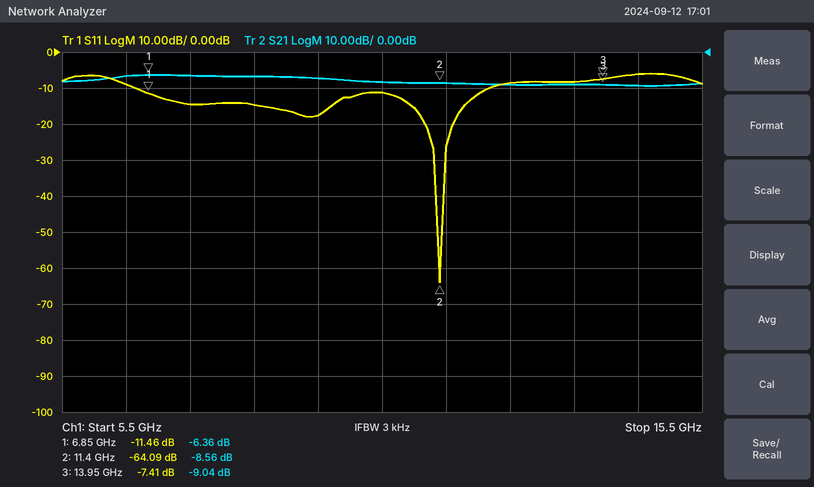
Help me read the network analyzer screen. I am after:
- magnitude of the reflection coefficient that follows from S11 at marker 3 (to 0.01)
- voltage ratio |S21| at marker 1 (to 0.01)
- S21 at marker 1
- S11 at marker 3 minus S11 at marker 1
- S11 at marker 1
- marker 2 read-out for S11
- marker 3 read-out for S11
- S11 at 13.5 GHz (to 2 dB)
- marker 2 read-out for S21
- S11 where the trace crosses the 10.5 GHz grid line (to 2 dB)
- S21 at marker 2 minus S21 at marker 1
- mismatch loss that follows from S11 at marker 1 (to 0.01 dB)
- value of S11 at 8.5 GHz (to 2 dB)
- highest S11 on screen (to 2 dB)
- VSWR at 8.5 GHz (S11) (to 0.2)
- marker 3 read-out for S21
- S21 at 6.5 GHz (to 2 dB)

0.43
0.48
-6.36 dB
4.05 dB
-11.46 dB
-64.09 dB
-7.41 dB
-8 dB
-8.56 dB
-12 dB
-2.20 dB
0.32 dB
-14 dB
-6 dB
1.4
-9.04 dB
-6 dB
